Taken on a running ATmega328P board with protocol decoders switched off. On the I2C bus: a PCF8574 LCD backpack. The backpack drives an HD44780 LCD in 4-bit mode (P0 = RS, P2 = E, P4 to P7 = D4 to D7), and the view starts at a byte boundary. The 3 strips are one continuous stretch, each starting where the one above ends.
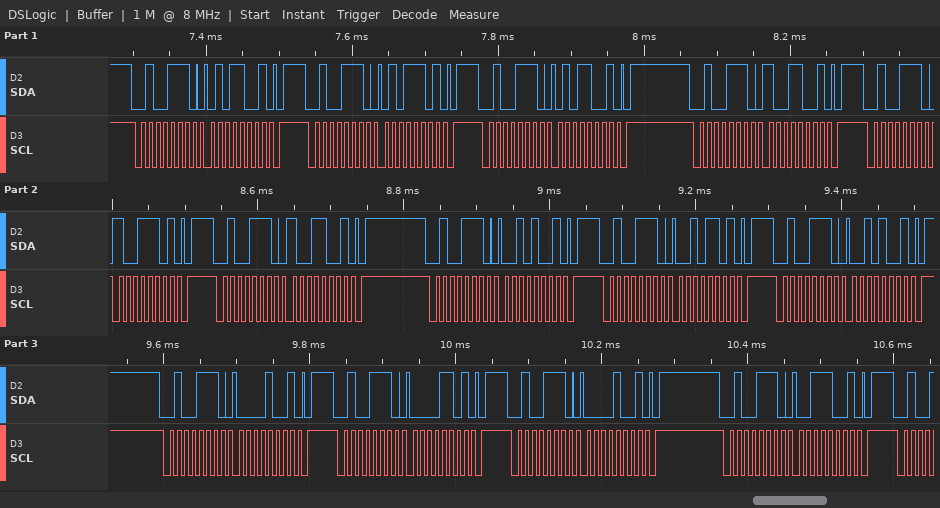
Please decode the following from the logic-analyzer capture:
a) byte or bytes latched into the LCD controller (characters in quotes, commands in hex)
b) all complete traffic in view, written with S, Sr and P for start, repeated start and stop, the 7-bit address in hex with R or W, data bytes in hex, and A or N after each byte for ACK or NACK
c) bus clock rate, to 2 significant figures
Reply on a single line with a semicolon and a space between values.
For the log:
'Y' ' '; S 27W A 59 A P S 27W A 5D A P S 27W A 59 A P S 27W A 99 A P S 27W A 9D A P S 27W A 99 A P S 27W A 29 A P S 27W A 2D A P S 27W A 29 A P S 27W A 09 A P S 27W A 0D A P S 27W A 09 A P S 27W A 39 A P; 100 kHz
